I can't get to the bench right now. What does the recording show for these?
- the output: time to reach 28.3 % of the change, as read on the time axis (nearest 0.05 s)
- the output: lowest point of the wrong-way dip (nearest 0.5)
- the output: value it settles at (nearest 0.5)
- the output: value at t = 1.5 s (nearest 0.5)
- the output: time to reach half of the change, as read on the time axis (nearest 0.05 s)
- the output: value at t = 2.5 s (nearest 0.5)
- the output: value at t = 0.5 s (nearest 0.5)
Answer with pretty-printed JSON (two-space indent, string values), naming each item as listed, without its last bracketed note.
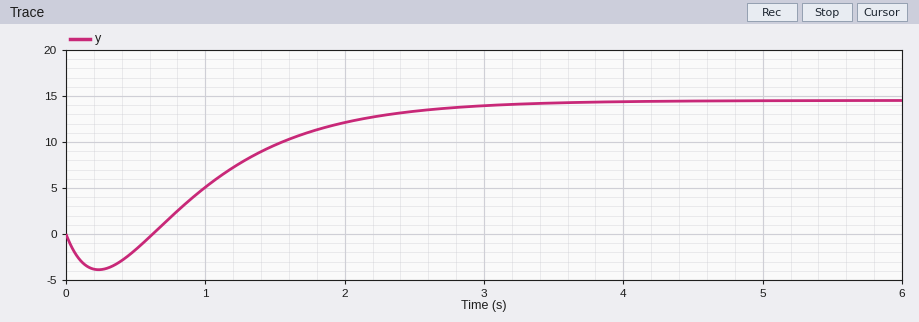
{
  "the output: time to reach 28.3 % of the change, as read on the time axis": "0.90 s",
  "the output: lowest point of the wrong-way dip": "-4.0",
  "the output: value it settles at": "14.5",
  "the output: value at t = 1.5 s": "9.5",
  "the output: time to reach half of the change, as read on the time axis": "1.20 s",
  "the output: value at t = 2.5 s": "13.5",
  "the output: value at t = 0.5 s": "-1.5"
}
